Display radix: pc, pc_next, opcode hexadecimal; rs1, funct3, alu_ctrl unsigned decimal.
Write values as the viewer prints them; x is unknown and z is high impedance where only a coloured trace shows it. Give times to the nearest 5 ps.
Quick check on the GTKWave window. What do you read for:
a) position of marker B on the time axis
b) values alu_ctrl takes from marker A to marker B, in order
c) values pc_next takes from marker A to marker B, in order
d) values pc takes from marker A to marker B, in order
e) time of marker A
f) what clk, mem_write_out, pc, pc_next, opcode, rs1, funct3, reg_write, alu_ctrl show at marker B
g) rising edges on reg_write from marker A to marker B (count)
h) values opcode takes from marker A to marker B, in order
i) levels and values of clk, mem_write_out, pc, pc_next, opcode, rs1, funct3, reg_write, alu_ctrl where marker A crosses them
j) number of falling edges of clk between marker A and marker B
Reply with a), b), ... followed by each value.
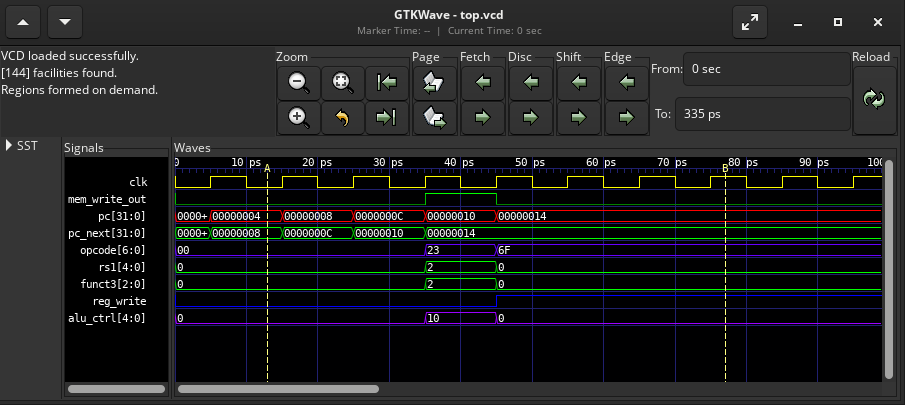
a) 75 ps
b) 0, 10, 0
c) 00000008, 0000000C, 00000010, 00000014
d) 00000004, 00000008, 0000000C, 00000010, 00000014
e) 15 ps
f) clk=1, mem_write_out=0, pc=00000014, pc_next=00000014, opcode=6F, rs1=0, funct3=0, reg_write=1, alu_ctrl=0
g) 1
h) 00, 23, 6F
i) clk=0, mem_write_out=0, pc=00000004, pc_next=00000008, opcode=00, rs1=0, funct3=0, reg_write=0, alu_ctrl=0
j) 6
